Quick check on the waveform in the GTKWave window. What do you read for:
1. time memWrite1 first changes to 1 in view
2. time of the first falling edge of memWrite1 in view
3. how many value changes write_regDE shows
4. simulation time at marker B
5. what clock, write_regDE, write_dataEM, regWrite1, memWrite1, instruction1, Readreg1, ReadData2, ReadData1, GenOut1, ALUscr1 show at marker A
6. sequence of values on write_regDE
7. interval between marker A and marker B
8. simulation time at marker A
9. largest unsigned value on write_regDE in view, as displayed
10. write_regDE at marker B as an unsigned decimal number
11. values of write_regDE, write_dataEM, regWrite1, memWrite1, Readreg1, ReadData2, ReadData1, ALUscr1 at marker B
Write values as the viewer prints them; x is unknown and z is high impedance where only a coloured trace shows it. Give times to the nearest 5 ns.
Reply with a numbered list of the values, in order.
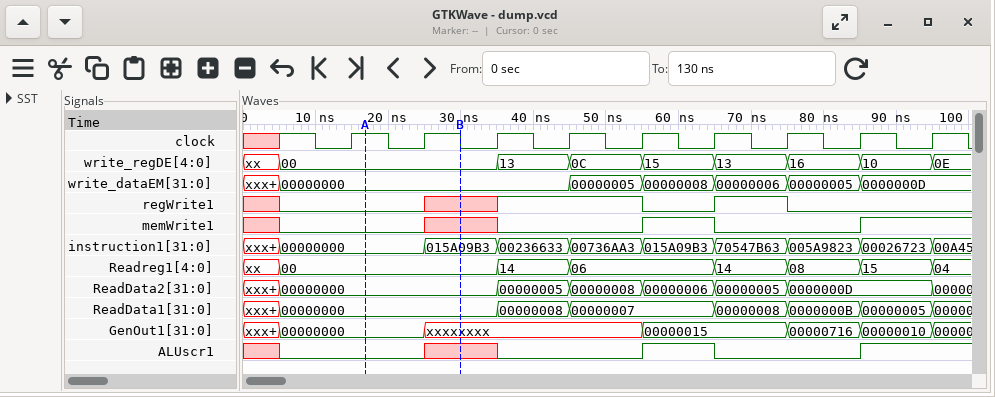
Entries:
1. 55 ns
2. 65 ns
3. 8
4. 30 ns
5. clock=1, write_regDE=00, write_dataEM=00000000, regWrite1=0, memWrite1=0, instruction1=00000000, Readreg1=00, ReadData2=00000000, ReadData1=00000000, GenOut1=00000000, ALUscr1=0
6. xx, 00, 13, 0C, 15, 13, 16, 10, 0E
7. 15 ns
8. 15 ns
9. 16
10. 0
11. write_regDE=00, write_dataEM=00000000, regWrite1=x, memWrite1=x, Readreg1=00, ReadData2=00000000, ReadData1=00000000, ALUscr1=x
